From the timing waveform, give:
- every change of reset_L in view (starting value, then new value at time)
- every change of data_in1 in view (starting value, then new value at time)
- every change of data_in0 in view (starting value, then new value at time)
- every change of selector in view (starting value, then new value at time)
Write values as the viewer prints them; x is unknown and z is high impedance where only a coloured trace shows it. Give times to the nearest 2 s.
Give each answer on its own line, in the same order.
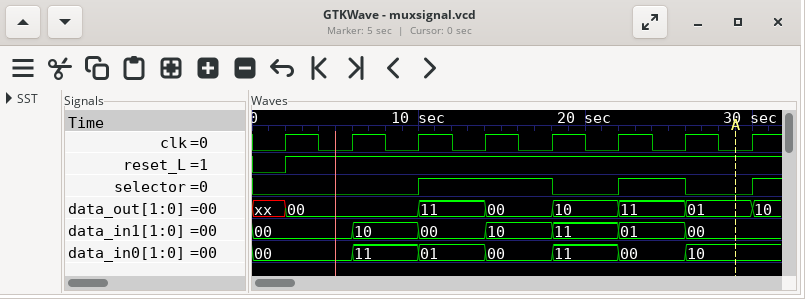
0, 1 at 2 s
00, 10 at 6 s, 00 at 10 s, 10 at 14 s, 11 at 18 s, 01 at 22 s, 00 at 26 s
00, 11 at 6 s, 01 at 10 s, 00 at 14 s, 11 at 18 s, 00 at 22 s, 10 at 26 s
0, 1 at 10 s, 0 at 18 s, 1 at 22 s, 0 at 26 s, 1 at 30 s
